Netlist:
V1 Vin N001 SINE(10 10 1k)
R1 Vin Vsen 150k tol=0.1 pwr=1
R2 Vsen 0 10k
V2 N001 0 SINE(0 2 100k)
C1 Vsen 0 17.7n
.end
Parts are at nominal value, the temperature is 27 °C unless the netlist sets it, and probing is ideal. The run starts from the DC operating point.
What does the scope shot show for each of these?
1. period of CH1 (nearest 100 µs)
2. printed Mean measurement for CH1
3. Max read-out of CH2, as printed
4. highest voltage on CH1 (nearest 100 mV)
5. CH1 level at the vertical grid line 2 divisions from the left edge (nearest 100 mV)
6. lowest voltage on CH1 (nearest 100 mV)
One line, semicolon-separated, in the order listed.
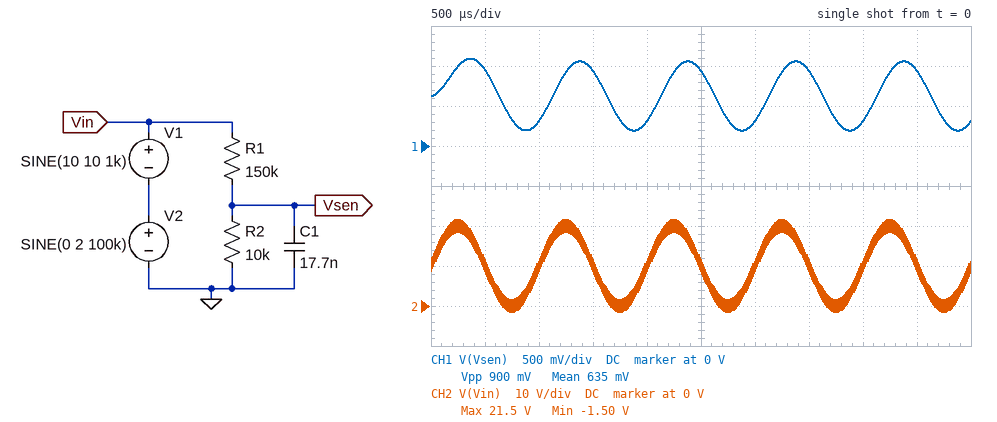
1.0 ms; 635 mV; 21.5 V; 1.1 V; 300 mV; 200 mV
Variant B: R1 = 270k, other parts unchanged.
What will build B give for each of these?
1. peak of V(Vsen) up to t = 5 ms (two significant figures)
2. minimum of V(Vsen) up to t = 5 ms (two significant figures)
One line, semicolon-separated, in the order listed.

620 mV; 110 mV
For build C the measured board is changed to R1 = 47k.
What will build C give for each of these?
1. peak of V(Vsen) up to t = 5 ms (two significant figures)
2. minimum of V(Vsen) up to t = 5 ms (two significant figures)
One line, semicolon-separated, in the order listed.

3.1 V; 460 mV
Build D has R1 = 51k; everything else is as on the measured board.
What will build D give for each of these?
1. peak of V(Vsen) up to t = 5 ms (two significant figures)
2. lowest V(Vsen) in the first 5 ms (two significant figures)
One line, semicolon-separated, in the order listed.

2.9 V; 440 mV
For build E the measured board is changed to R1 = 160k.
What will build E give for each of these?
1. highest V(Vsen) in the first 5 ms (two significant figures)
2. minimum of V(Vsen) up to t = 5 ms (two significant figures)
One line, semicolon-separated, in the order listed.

1.0 V; 180 mV
